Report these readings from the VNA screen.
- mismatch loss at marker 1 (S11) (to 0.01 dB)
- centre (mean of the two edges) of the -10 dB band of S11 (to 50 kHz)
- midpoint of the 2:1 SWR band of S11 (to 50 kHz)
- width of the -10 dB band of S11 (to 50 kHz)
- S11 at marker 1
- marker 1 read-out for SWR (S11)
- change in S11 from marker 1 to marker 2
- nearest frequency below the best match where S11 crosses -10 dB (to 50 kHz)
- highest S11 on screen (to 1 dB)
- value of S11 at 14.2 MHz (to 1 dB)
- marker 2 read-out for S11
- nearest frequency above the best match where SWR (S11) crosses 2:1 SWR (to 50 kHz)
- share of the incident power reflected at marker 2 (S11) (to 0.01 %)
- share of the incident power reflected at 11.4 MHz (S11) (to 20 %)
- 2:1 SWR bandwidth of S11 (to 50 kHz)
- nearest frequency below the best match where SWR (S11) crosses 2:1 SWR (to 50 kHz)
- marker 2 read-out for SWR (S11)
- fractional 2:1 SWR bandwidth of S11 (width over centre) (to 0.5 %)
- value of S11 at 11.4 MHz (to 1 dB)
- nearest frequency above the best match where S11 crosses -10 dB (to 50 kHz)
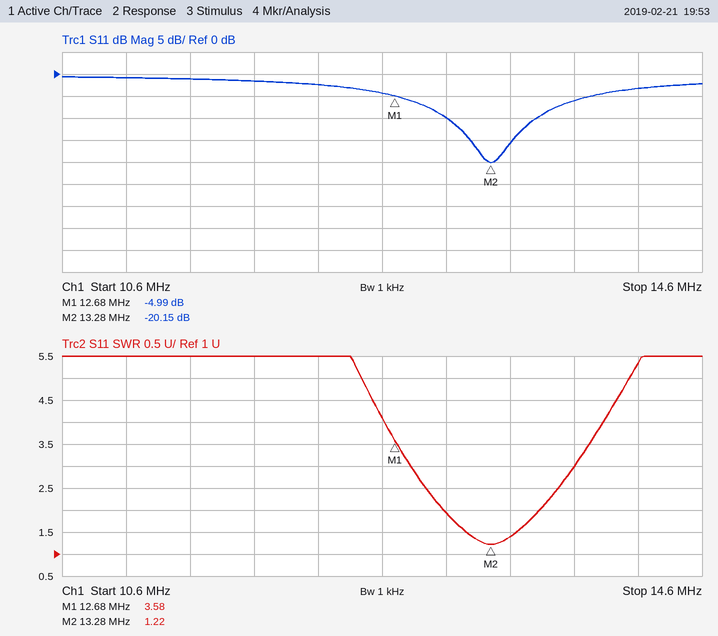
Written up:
1.66 dB
13.30 MHz
13.30 MHz
550 kHz
-4.99 dB
3.58
-15.16 dB
13.00 MHz
-1 dB
-3 dB
-20.15 dB
13.60 MHz
0.97 %
80 %
600 kHz
13.00 MHz
1.22
4.5 %
-1 dB
13.55 MHz
